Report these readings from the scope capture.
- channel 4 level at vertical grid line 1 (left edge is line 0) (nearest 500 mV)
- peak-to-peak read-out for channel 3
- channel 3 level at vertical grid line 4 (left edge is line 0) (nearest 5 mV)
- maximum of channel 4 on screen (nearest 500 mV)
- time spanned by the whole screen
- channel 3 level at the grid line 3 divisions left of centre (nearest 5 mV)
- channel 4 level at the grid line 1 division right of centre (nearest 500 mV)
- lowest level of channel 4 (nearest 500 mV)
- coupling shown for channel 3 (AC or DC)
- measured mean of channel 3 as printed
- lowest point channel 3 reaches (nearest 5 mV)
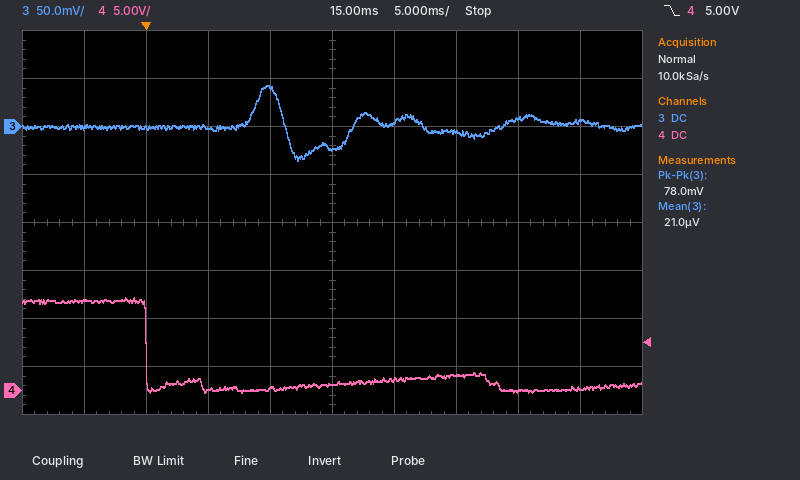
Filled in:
9.5 V
78.0 mV
40 mV
9.5 V
50 ms
0 mV
1.0 V
0.0 V
DC
21.0 µV
-35 mV
